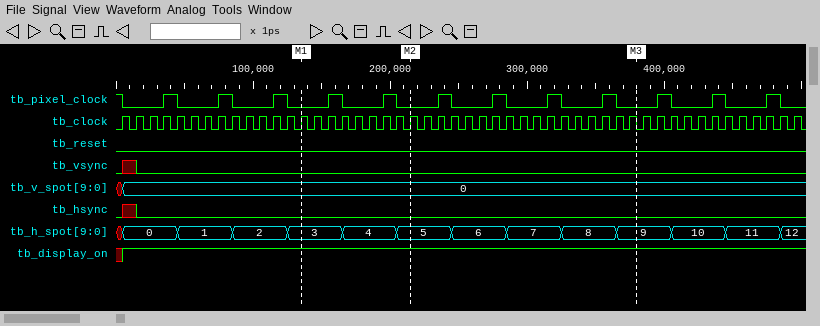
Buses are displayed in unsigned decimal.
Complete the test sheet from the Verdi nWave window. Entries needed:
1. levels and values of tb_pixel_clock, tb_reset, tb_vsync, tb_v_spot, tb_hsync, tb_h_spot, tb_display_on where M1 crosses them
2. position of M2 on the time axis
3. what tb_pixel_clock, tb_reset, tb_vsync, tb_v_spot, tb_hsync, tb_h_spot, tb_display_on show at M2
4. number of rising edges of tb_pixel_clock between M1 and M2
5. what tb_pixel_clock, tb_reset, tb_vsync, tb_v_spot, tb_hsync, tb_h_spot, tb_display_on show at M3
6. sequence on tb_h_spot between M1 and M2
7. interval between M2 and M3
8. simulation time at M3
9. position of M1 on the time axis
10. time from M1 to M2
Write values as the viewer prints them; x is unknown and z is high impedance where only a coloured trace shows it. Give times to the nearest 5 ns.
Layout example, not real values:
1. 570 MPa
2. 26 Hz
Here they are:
1. tb_pixel_clock=0, tb_reset=0, tb_vsync=0, tb_v_spot=0, tb_hsync=0, tb_h_spot=3, tb_display_on=1
2. 215 ns
3. tb_pixel_clock=0, tb_reset=0, tb_vsync=0, tb_v_spot=0, tb_hsync=0, tb_h_spot=5, tb_display_on=1
4. 2
5. tb_pixel_clock=0, tb_reset=0, tb_vsync=0, tb_v_spot=0, tb_hsync=0, tb_h_spot=9, tb_display_on=1
6. 3, 4, 5
7. 165 ns
8. 380 ns
9. 135 ns
10. 80 ns
